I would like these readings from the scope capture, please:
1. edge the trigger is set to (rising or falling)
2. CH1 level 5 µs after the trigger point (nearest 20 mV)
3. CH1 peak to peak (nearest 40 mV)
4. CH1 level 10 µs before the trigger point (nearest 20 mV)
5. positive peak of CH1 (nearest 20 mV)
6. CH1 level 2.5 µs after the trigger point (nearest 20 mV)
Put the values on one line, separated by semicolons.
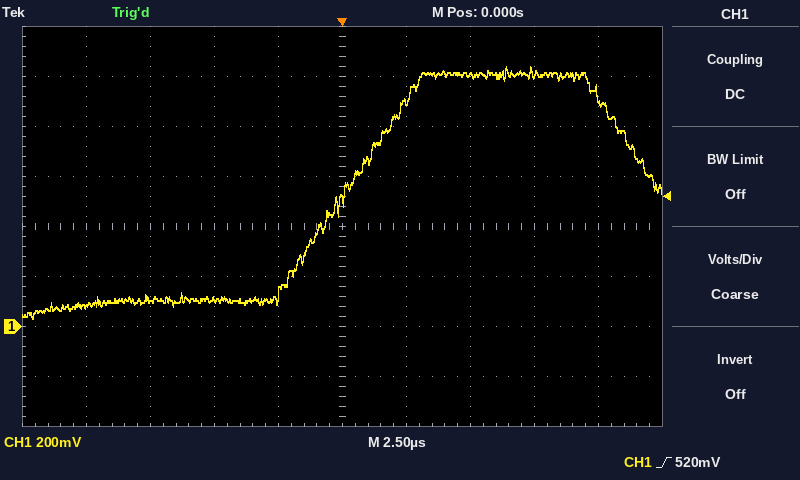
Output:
rising; 1.00 V; 1.00 V; 80 mV; 1.04 V; 900 mV
